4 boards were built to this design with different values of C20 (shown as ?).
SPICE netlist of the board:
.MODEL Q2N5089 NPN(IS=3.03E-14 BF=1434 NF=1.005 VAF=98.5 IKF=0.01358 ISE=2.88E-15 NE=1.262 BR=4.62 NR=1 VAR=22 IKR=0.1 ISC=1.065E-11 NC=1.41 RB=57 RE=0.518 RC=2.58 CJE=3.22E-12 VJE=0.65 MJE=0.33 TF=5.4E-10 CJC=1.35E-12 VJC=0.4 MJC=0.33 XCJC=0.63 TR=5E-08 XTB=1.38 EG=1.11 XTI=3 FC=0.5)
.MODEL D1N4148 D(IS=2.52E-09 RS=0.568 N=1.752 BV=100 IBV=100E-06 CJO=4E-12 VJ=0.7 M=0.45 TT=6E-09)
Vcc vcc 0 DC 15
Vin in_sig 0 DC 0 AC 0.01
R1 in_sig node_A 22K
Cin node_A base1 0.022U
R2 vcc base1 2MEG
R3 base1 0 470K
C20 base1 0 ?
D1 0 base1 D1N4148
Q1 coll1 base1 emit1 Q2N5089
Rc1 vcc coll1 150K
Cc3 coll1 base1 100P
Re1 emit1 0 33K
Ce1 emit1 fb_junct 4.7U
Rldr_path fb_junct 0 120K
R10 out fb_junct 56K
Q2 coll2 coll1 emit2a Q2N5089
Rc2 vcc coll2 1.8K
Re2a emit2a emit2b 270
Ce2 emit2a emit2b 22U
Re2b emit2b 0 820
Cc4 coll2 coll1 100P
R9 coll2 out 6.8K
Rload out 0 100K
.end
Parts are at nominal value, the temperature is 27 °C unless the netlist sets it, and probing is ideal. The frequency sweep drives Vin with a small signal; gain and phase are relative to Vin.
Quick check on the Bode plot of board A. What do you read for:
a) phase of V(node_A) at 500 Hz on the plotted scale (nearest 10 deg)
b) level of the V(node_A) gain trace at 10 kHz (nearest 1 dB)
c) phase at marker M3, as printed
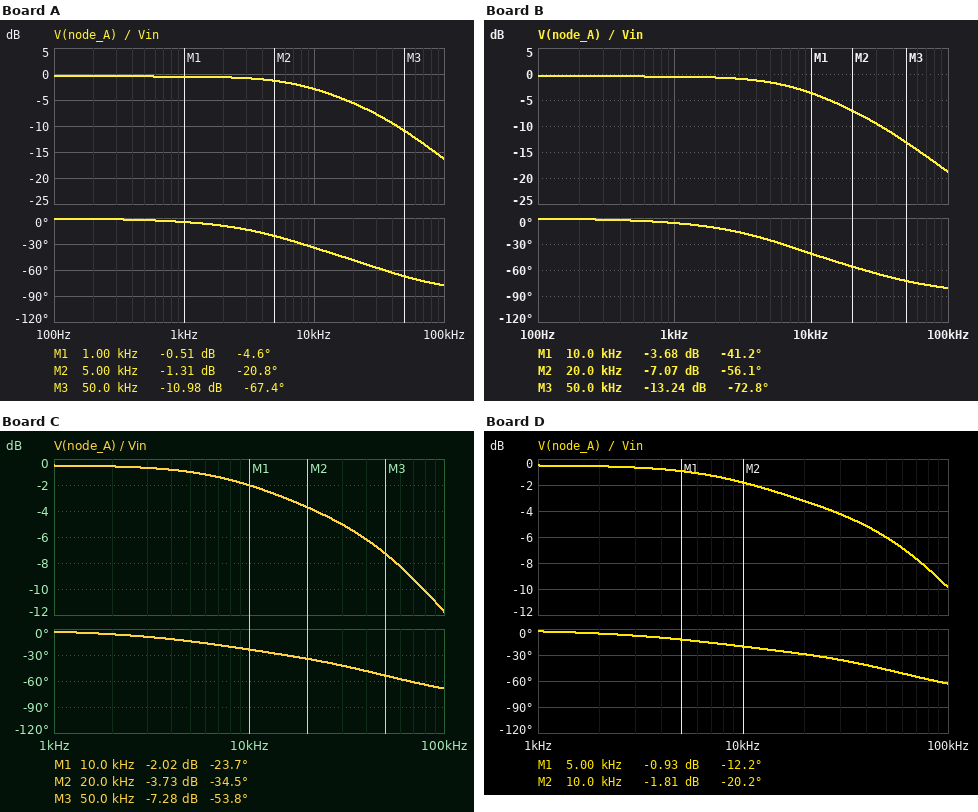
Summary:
0 deg
-3 dB
-67.4 deg
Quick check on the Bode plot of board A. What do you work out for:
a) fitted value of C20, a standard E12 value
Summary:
390 pF
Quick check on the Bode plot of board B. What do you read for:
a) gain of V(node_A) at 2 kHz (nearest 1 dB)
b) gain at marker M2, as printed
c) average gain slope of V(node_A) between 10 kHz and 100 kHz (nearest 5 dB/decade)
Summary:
-1 dB
-7.07 dB
-15 dB/decade
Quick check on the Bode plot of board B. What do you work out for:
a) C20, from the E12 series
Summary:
560 pF
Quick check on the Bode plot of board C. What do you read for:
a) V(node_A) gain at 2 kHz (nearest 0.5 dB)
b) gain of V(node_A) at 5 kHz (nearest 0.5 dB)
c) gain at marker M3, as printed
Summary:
-0.5 dB
-1.0 dB
-7.28 dB
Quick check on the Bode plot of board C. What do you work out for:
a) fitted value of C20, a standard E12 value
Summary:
180 pF
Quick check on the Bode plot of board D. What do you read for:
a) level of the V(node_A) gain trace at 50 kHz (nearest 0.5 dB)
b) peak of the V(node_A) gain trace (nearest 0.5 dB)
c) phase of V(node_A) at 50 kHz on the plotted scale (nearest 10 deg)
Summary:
-6.0 dB
-0.5 dB
-50 deg
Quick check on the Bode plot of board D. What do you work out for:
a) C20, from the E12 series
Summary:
120 pF
